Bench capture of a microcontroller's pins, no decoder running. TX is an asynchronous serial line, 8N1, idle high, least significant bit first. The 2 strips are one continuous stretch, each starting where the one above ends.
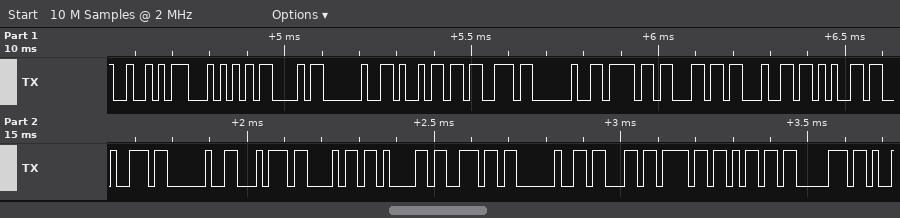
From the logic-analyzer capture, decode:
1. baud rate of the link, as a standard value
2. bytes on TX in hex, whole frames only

57600 baud
0x52 0x54 0x43 0x20 0x69 0x73 0x20 0x6F 0x6C 0x64 0x65 0x72 0x20 0x74 0x68 0x61 0x6E 0x20 0x63 0x6F 0x6D 0x70
